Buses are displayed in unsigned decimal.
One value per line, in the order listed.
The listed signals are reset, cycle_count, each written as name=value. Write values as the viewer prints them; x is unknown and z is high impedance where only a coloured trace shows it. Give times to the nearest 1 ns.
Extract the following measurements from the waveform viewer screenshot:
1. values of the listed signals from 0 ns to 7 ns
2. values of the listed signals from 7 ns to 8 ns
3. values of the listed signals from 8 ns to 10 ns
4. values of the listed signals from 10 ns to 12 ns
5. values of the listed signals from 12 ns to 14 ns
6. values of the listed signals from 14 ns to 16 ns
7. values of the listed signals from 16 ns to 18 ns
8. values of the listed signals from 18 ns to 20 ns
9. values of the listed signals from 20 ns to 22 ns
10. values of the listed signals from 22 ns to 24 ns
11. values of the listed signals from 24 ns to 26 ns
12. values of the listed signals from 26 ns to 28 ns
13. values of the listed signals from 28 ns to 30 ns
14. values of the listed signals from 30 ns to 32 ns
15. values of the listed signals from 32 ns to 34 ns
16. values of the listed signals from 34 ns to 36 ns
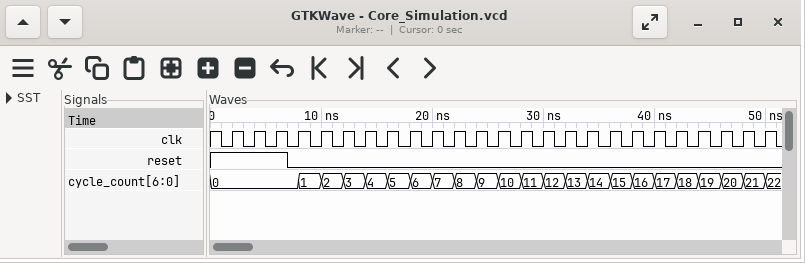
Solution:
reset=1, cycle_count=0
reset=0, cycle_count=0
reset=0, cycle_count=1
reset=0, cycle_count=2
reset=0, cycle_count=3
reset=0, cycle_count=4
reset=0, cycle_count=5
reset=0, cycle_count=6
reset=0, cycle_count=7
reset=0, cycle_count=8
reset=0, cycle_count=9
reset=0, cycle_count=10
reset=0, cycle_count=11
reset=0, cycle_count=12
reset=0, cycle_count=13
reset=0, cycle_count=14
